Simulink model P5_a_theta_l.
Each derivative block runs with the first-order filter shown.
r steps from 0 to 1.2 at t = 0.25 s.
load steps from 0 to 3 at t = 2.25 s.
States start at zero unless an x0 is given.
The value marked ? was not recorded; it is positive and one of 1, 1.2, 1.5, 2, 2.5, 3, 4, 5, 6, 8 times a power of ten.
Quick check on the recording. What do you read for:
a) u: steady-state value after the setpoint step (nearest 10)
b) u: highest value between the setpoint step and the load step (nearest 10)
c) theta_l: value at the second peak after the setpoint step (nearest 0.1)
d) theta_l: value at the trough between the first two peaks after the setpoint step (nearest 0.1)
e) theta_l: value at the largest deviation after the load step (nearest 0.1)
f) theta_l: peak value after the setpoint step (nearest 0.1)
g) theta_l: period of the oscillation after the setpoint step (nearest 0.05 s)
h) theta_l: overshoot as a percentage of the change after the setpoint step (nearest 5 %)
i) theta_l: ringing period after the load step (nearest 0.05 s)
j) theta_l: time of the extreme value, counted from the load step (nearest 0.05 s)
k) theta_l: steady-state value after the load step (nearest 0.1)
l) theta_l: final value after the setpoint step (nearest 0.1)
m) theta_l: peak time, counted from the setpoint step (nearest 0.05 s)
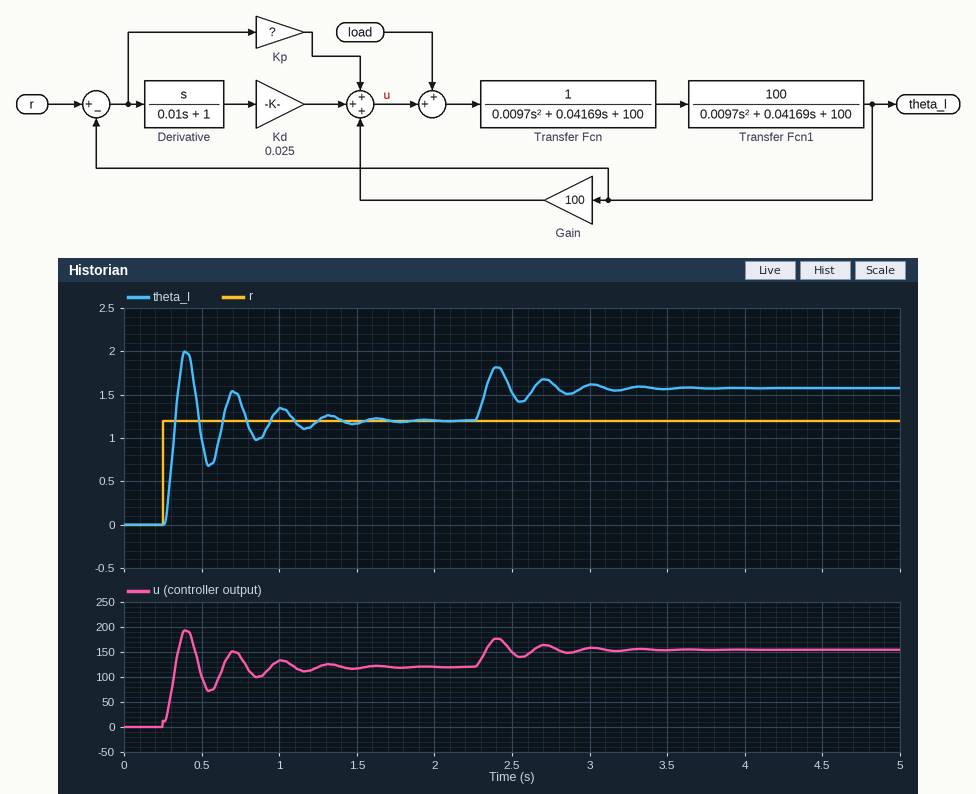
120
190
1.5
0.7
1.8
2.0
0.30 s
65 %
0.30 s
0.15 s
1.6
1.2
0.15 s
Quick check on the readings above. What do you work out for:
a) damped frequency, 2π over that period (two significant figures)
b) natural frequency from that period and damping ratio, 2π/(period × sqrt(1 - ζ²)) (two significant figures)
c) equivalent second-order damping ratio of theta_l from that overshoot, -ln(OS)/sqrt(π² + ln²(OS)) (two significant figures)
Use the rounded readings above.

21 rad/s
21 rad/s
0.14
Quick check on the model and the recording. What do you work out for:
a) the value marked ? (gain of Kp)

8
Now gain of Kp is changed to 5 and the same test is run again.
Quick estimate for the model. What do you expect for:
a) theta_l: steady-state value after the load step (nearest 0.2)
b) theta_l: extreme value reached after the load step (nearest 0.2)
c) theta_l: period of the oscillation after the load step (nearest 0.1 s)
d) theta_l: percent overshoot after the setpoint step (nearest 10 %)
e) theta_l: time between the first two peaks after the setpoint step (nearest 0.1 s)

1.8
2.2
0.4 s
60 %
0.4 s
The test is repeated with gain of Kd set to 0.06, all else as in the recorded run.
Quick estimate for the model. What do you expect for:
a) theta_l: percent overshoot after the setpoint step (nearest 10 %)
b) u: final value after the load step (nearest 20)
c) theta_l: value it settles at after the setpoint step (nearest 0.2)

60 %
160
1.2
